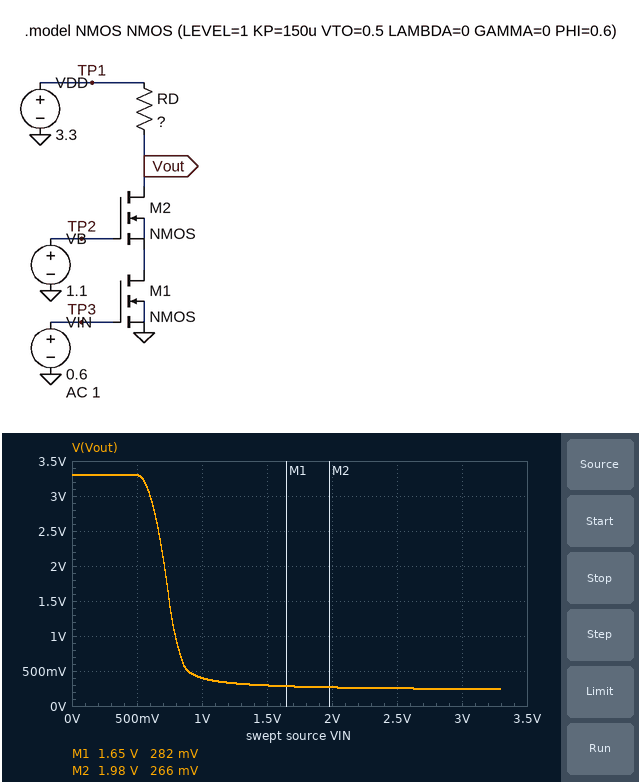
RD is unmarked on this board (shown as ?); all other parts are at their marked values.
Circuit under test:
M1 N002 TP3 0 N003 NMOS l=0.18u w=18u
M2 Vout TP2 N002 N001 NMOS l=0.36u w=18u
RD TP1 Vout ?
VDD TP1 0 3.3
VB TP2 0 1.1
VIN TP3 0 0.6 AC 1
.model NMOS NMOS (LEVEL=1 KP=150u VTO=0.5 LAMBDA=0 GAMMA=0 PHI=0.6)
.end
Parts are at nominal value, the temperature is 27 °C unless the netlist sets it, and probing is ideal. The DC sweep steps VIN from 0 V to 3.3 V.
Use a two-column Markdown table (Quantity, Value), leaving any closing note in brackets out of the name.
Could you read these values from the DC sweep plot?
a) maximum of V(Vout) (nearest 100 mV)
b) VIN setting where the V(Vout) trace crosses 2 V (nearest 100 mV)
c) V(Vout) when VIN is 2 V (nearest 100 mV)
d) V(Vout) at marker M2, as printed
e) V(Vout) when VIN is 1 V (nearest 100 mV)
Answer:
| Quantity | Value |
|---|---|
| maximum of V(Vout) | 3.3 V |
| VIN setting where the V(Vout) trace crosses 2 V | 700 mV |
| V(Vout) when VIN is 2 V | 300 mV |
| V(Vout) at marker M2, as printed | 266 mV |
| V(Vout) when VIN is 1 V | 400 mV |
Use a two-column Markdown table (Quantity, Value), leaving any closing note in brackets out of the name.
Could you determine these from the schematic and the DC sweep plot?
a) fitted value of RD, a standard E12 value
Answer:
| Quantity | Value |
|---|---|
| fitted value of RD, a standard E12 value | 3.9 kΩ |
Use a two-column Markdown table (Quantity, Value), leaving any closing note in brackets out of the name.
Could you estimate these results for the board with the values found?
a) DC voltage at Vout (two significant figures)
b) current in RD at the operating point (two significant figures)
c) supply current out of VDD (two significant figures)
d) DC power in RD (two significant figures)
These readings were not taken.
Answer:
| Quantity | Value |
|---|---|
| DC voltage at Vout | 3.0 V |
| current in RD at the operating point | 75 µA |
| supply current out of VDD | 75 µA |
| DC power in RD | 22 µW |
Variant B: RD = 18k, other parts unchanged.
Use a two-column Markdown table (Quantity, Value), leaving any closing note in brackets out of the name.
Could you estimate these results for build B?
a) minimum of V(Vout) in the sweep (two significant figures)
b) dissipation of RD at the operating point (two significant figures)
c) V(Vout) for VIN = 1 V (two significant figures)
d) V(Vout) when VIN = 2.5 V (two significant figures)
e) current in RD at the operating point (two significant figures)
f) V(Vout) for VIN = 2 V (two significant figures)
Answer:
| Quantity | Value |
|---|---|
| minimum of V(Vout) in the sweep | 46 mV |
| dissipation of RD at the operating point | 100 µW |
| V(Vout) for VIN = 1 V | 68 mV |
| V(Vout) when VIN = 2.5 V | 48 mV |
| current in RD at the operating point | 75 µA |
| V(Vout) for VIN = 2 V | 50 mV |
